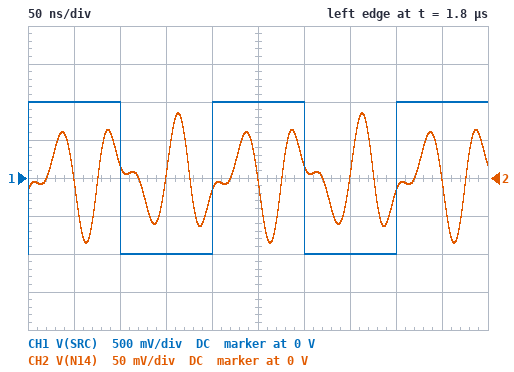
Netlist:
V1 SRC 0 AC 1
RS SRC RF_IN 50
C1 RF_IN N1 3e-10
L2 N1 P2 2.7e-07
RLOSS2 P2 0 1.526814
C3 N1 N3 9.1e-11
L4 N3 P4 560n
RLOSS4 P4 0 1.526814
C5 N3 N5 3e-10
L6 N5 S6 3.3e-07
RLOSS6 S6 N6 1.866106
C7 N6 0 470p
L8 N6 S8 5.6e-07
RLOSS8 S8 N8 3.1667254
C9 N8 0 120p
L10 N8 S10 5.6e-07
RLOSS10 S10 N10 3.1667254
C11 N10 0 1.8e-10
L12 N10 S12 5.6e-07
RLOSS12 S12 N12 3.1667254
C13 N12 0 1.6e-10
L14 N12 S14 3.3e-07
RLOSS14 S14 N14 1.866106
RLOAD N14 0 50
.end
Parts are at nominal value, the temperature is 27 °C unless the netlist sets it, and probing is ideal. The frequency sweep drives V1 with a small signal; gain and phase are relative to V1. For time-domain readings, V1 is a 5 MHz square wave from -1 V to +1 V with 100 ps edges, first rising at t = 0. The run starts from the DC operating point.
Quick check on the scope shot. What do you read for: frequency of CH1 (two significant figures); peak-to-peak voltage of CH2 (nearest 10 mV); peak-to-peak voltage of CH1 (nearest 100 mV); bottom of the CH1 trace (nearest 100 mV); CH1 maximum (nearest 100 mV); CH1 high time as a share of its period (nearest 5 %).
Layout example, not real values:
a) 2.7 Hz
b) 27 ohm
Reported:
a) 5.0 MHz
b) 170 mV
c) 2.0 V
d) -1.0 V
e) 1.0 V
f) 50 %
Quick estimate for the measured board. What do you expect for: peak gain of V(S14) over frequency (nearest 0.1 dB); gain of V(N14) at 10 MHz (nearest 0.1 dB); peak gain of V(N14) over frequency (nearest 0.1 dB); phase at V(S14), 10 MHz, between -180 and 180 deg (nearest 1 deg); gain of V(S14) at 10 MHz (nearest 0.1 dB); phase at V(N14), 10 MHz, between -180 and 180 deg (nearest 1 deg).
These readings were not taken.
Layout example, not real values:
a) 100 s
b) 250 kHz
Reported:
a) -15.5 dB
b) -22.3 dB
c) -15.8 dB
d) 152 deg
e) -22.0 dB
f) 152 deg
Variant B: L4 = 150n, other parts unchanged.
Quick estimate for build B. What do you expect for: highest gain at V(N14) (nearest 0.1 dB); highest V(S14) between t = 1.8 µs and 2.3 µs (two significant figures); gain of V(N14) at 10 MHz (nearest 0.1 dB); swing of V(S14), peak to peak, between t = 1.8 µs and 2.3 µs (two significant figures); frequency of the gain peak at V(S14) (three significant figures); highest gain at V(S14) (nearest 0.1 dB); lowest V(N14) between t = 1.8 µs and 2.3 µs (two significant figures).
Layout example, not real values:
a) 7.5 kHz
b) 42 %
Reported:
a) -14.1 dB
b) 60 mV
c) -41.5 dB
d) 120 mV
e) 17.2 MHz
f) -13.7 dB
g) -58 mV
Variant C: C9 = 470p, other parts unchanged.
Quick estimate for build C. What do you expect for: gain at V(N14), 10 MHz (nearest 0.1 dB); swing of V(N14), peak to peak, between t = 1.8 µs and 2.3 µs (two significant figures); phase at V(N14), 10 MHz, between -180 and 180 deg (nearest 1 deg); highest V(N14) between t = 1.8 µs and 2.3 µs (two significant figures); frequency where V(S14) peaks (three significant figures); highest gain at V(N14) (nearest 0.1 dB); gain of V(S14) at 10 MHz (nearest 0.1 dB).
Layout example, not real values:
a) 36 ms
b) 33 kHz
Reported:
a) -21.8 dB
b) 190 mV
c) 95 deg
d) 93 mV
e) 14.6 MHz
f) -13.7 dB
g) -21.5 dB
